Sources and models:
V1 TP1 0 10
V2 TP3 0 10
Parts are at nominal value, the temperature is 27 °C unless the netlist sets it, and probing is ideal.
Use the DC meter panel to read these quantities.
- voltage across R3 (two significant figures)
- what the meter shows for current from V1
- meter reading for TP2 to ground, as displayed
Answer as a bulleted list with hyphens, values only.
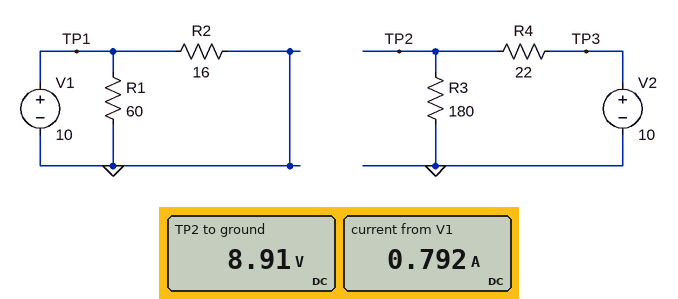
- 8.9 V
- 0.792 A
- 8.91 V
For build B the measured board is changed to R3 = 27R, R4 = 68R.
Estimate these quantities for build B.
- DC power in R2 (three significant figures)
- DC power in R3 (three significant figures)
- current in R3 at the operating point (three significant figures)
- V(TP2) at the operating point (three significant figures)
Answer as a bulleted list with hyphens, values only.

- 6.25 W
- 299 mW
- 105 mA
- 2.84 V
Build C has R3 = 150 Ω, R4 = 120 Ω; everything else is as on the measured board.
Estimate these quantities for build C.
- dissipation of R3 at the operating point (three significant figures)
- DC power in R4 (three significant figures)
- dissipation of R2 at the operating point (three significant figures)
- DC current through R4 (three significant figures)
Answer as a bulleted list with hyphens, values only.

- 206 mW
- 165 mW
- 6.25 W
- 37.0 mA
